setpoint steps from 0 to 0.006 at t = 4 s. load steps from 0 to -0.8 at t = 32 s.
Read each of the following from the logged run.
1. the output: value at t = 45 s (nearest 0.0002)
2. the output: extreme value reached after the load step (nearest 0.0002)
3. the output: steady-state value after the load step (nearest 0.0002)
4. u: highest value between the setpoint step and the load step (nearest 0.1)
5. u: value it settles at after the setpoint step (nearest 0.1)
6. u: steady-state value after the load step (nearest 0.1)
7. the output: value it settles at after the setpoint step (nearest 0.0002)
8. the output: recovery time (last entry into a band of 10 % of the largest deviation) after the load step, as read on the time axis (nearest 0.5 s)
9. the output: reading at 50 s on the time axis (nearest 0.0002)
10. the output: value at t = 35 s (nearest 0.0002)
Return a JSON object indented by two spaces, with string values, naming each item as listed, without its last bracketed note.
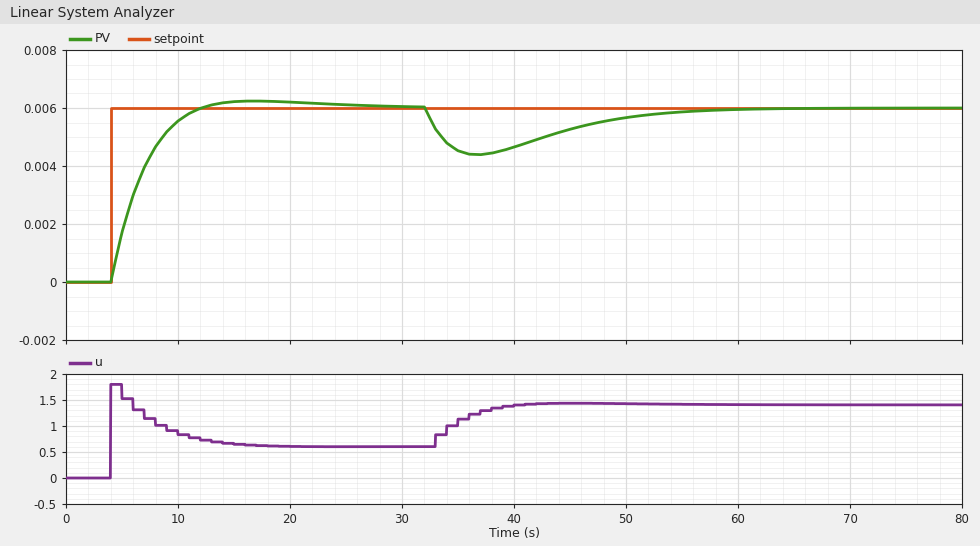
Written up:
{
  "the output: value at t = 45 s": "0.0052",
  "the output: extreme value reached after the load step": "0.0044",
  "the output: steady-state value after the load step": "0.0060",
  "u: highest value between the setpoint step and the load step": "1.8",
  "u: value it settles at after the setpoint step": "0.6",
  "u: steady-state value after the load step": "1.4",
  "the output: value it settles at after the setpoint step": "0.0060",
  "the output: recovery time (last entry into a band of 10 % of the largest deviation) after the load step, as read on the time axis": "54.0 s",
  "the output: reading at 50 s on the time axis": "0.0056",
  "the output: value at t = 35 s": "0.0046"
}
